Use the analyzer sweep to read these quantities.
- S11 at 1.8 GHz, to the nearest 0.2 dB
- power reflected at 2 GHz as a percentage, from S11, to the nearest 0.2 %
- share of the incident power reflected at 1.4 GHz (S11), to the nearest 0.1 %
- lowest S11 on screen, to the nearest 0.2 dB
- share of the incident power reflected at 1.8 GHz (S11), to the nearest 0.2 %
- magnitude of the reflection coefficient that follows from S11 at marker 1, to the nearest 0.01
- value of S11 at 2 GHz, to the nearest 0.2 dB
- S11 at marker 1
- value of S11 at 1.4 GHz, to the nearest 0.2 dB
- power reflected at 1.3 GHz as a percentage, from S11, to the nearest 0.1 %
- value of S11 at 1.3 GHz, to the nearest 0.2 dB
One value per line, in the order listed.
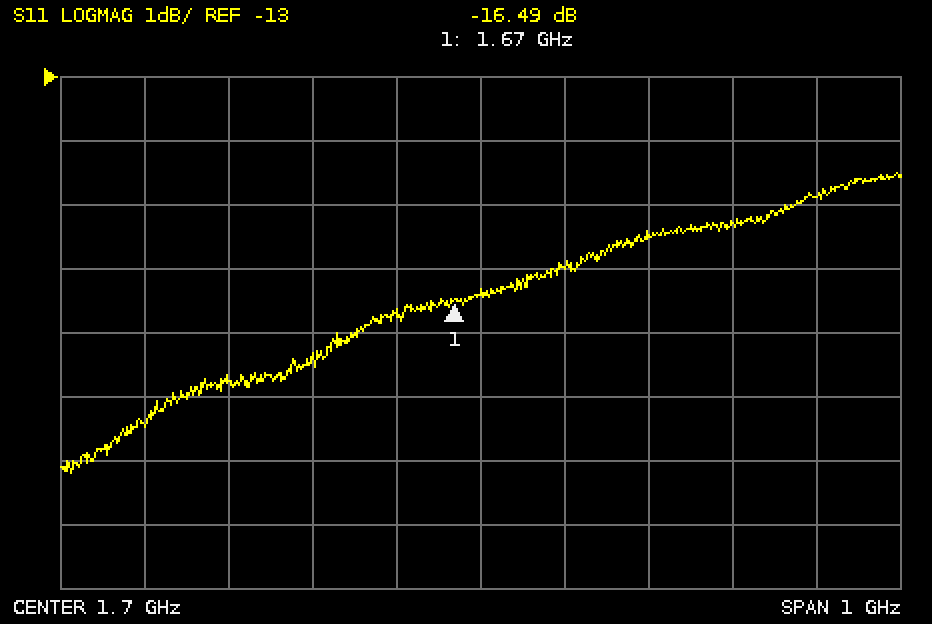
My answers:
-16.0 dB
3.0 %
1.7 %
-19.2 dB
2.6 %
0.15
-15.2 dB
-16.49 dB
-17.8 dB
1.4 %
-18.4 dB
